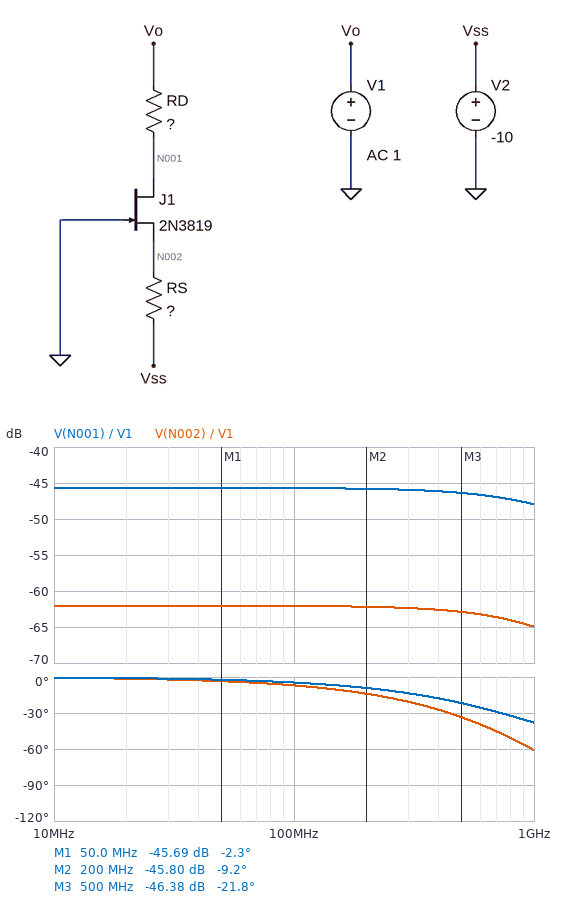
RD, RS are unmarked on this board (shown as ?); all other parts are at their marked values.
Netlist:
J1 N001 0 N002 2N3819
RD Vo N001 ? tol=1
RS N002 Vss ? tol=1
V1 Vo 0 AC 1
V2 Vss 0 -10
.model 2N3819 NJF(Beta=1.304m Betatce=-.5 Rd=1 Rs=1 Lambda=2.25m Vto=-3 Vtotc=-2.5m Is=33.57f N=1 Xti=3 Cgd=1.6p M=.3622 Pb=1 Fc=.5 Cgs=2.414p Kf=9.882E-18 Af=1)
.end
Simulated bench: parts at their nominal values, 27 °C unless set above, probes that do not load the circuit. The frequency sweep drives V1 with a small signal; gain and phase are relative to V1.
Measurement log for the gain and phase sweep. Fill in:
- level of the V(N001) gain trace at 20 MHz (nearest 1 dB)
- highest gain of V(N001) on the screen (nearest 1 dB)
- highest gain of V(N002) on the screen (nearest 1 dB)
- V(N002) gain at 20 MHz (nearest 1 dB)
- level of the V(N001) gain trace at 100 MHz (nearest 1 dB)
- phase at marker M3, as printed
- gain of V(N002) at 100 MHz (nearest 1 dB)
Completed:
-46 dB
-46 dB
-62 dB
-62 dB
-46 dB
-21.8 deg
-62 dB
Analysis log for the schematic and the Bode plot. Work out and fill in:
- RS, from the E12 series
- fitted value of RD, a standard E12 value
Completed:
5.6 kΩ
10 kΩ
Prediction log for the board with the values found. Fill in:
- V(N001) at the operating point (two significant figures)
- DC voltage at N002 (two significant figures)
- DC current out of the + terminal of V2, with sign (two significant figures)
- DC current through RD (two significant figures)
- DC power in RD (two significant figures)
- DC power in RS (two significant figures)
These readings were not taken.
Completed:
-590 mV
-630 mV
-1.7 mA
59 µA
35 µW
16 mW
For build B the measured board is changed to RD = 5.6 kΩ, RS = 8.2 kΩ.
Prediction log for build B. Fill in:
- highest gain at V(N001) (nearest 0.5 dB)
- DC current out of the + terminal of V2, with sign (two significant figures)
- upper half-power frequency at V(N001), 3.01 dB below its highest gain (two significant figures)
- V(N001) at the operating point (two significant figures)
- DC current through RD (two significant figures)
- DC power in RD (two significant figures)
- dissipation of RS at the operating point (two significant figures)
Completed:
-39.0 dB
-1.1 mA
940 MHz
-580 mV
100 µA
61 µW
11 mW
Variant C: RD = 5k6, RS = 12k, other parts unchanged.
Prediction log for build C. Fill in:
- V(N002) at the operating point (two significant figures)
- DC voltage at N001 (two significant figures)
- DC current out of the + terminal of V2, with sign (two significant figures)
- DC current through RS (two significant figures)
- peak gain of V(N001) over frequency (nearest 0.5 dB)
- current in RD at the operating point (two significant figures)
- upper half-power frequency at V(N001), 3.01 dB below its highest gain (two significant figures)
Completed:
-610 mV
-580 mV
-780 µA
780 µA
-37.0 dB
100 µA
710 MHz
